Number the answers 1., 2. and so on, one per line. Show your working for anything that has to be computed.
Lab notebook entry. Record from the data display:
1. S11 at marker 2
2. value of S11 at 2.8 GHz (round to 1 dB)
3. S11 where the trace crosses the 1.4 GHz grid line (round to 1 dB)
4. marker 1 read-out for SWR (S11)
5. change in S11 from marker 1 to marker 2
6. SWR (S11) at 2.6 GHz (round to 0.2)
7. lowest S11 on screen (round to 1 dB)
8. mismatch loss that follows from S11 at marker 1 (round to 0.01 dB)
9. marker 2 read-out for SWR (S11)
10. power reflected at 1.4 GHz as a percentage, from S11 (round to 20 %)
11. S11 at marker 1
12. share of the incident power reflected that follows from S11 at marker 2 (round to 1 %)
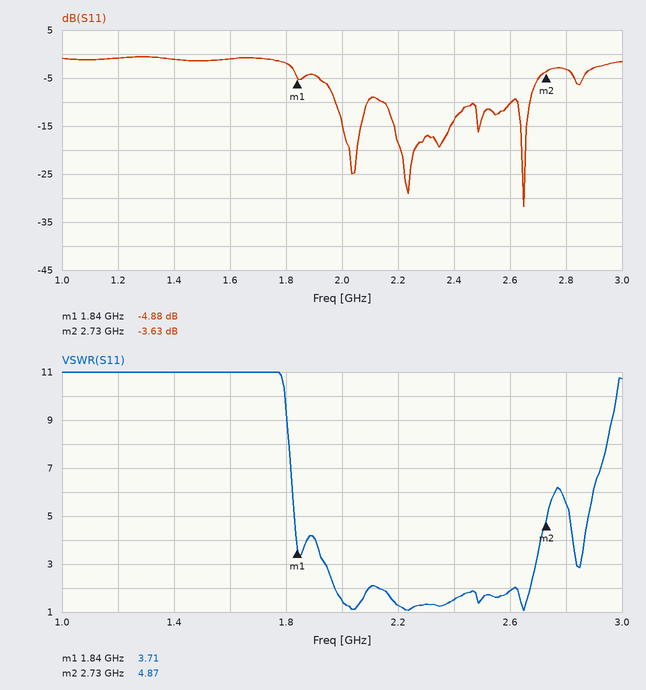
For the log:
1. -3.63 dB
2. -3 dB
3. -1 dB
4. 3.71
5. -3.63 − (-4.88) = 1.25 dB
6. 1.8
7. -32 dB
8. −10 log10(1 − 10^(-4.88/10)) ≈ 1.71 dB
9. 4.87
10. 10^(-1/10) ≈ 79.4 %, so 80 % to the nearest 20 %
11. -4.88 dB
12. 10^(-3.63/10) ≈ 43 %
